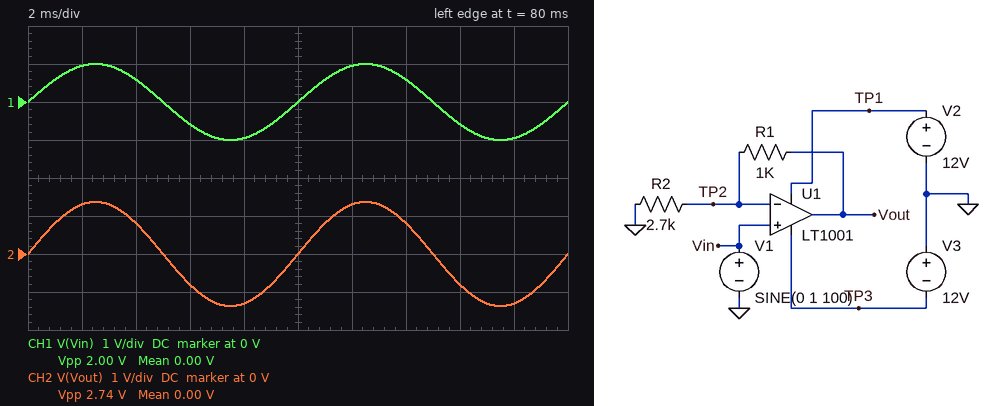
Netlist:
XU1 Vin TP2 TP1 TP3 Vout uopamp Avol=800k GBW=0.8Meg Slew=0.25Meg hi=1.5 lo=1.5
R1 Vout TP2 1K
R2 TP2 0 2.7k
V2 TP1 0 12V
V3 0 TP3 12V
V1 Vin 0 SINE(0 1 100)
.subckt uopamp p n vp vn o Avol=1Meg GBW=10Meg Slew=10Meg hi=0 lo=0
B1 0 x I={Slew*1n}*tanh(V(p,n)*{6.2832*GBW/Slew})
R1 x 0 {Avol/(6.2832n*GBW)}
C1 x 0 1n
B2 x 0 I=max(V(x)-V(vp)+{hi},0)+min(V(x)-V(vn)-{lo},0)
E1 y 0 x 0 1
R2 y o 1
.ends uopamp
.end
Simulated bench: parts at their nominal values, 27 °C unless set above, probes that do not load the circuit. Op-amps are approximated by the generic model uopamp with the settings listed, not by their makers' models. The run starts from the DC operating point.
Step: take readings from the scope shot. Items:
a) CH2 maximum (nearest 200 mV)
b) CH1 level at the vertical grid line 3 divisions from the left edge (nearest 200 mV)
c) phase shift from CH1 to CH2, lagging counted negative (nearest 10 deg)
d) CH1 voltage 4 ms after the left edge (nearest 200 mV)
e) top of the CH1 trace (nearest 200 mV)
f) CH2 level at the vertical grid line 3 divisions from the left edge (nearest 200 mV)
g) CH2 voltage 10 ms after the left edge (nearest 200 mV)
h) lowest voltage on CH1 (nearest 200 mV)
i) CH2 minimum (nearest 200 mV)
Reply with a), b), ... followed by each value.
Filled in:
a) 1.4 V
b) -600 mV
c) 0 deg
d) 600 mV
e) 1.0 V
f) -800 mV
g) 0 V
h) -1.0 V
i) -1.4 V
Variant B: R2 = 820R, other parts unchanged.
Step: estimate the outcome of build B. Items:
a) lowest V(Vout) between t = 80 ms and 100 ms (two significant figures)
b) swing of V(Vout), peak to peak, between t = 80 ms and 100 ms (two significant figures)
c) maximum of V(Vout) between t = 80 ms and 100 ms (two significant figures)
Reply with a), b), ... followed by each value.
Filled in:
a) -2.2 V
b) 4.4 V
c) 2.2 V
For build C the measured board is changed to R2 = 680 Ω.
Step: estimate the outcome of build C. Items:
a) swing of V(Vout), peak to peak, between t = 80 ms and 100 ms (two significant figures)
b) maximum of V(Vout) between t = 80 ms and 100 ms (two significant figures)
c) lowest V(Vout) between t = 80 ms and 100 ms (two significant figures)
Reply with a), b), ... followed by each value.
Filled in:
a) 4.9 V
b) 2.5 V
c) -2.5 V
